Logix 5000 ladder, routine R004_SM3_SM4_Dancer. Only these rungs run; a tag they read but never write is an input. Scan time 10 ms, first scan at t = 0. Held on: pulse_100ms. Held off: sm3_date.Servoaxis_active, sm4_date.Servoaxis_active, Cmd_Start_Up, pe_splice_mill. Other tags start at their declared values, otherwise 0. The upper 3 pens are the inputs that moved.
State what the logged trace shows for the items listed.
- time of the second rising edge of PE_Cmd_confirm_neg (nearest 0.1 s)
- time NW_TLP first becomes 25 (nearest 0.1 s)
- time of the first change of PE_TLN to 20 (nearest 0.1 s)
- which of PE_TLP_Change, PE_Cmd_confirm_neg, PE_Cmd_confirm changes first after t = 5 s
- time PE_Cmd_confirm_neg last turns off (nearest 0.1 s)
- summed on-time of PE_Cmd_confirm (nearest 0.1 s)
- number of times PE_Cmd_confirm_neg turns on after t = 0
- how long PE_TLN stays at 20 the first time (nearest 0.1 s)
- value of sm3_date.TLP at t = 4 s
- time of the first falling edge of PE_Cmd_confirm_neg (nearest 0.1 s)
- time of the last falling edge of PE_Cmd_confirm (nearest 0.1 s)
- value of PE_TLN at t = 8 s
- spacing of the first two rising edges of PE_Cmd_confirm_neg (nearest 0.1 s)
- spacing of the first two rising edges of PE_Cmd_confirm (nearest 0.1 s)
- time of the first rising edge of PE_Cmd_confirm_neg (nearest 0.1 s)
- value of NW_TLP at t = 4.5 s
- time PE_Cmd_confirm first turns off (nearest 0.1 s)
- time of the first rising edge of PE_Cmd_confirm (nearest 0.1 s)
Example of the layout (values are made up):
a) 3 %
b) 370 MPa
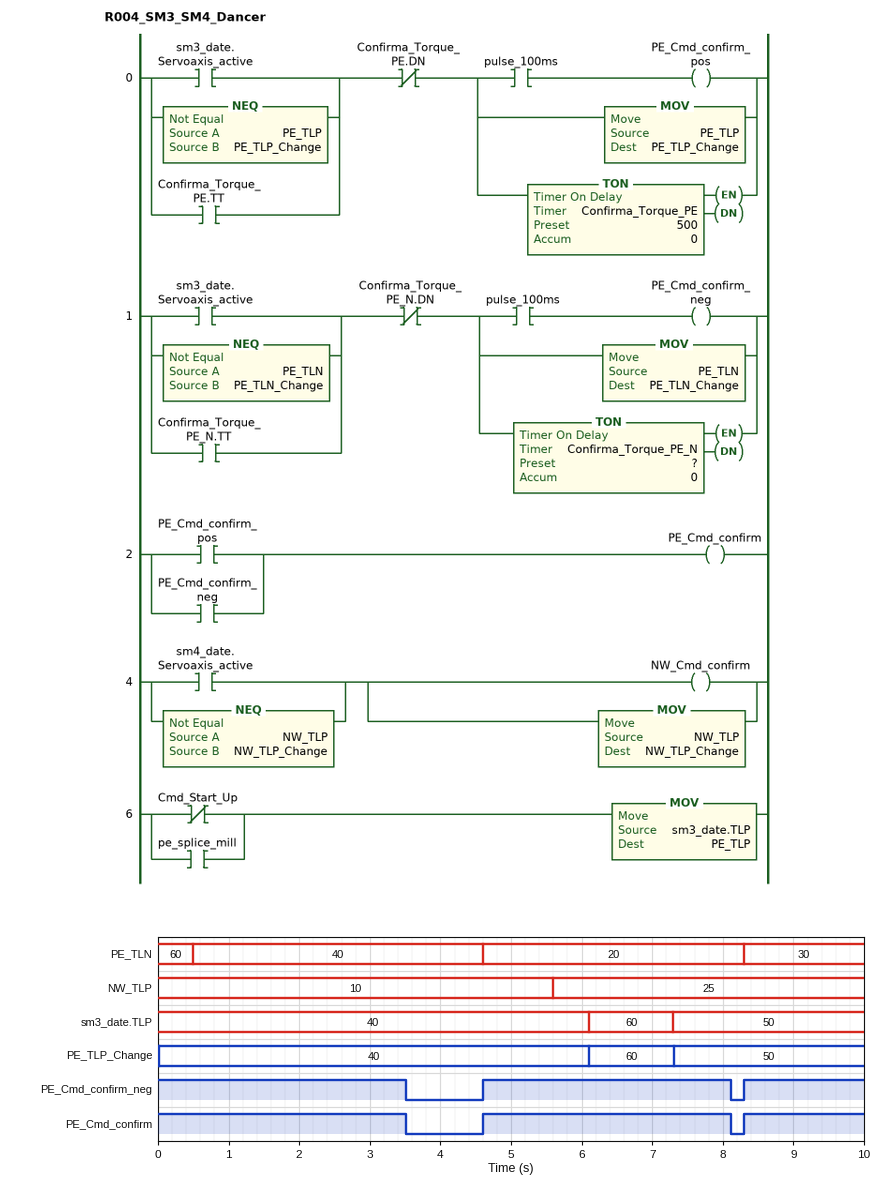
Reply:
a) 8.3 s
b) 5.6 s
c) 4.6 s
d) PE_TLP_Change
e) 8.1 s
f) 8.7 s
g) 2
h) 3.7 s
i) 40
j) 3.5 s
k) 8.1 s
l) 20
m) 3.7 s
n) 3.7 s
o) 4.6 s
p) 10
q) 3.5 s
r) 4.6 s
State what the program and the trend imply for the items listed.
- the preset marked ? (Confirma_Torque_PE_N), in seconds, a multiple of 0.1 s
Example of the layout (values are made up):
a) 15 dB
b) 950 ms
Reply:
a) 3.5 s
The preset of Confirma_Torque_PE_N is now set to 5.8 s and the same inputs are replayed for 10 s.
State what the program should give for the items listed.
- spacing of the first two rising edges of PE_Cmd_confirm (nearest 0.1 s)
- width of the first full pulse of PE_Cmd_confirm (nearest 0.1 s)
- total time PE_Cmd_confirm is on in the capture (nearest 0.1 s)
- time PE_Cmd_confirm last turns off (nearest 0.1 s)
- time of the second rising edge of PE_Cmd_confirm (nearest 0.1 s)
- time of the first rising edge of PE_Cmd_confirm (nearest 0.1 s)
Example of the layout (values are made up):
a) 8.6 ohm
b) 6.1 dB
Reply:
a) 1.2 s
b) 0.5 s
c) 8.5 s
d) 7.8 s
e) 7.3 s
f) 6.1 s
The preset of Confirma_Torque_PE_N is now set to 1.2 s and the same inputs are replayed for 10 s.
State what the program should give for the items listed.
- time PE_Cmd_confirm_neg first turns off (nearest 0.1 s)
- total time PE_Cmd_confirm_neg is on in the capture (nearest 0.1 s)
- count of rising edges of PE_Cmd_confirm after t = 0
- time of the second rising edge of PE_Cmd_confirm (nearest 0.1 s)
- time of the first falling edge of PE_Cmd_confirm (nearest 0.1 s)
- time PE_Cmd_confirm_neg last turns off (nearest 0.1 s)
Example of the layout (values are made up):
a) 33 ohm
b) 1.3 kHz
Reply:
a) 1.2 s
b) 3.6 s
c) 4
d) 6.1 s
e) 1.2 s
f) 9.5 s
